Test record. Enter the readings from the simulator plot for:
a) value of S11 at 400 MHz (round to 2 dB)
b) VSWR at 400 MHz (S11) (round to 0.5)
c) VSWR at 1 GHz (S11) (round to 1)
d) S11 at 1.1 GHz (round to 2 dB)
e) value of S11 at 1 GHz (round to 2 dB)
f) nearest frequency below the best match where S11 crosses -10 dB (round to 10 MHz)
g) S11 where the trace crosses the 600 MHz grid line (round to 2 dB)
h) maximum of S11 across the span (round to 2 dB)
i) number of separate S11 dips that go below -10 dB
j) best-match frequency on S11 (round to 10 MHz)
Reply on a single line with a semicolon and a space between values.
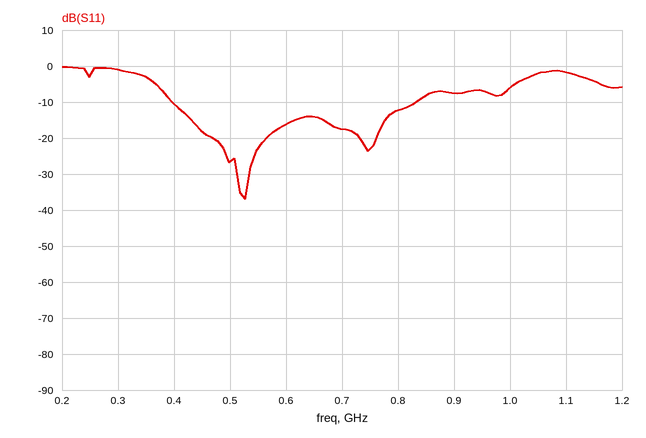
-10 dB; 2.0; 3; -2 dB; -6 dB; 400 MHz; -16 dB; 0 dB; 2; 530 MHz
